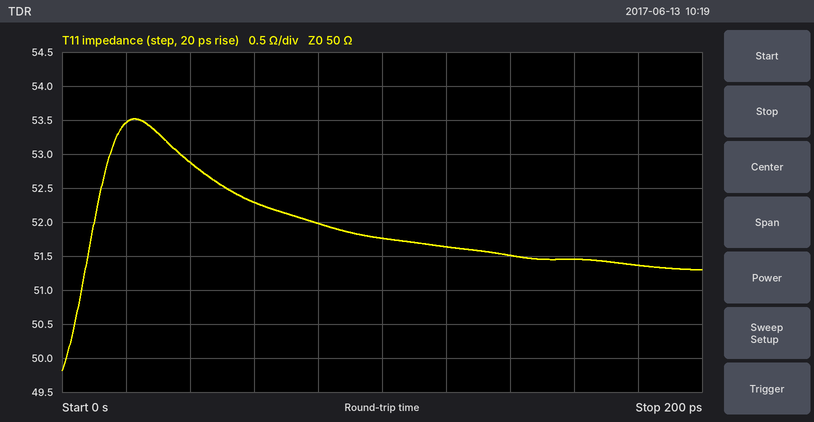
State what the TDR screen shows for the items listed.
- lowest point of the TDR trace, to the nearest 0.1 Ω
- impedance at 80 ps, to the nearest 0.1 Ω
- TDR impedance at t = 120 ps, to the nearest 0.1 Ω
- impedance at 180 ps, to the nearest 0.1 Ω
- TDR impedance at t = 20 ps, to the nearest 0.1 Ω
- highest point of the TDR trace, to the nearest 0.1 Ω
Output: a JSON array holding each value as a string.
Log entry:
["49.8 Ω", "52.0 Ω", "51.6 Ω", "51.4 Ω", "53.5 Ω", "53.5 Ω"]
